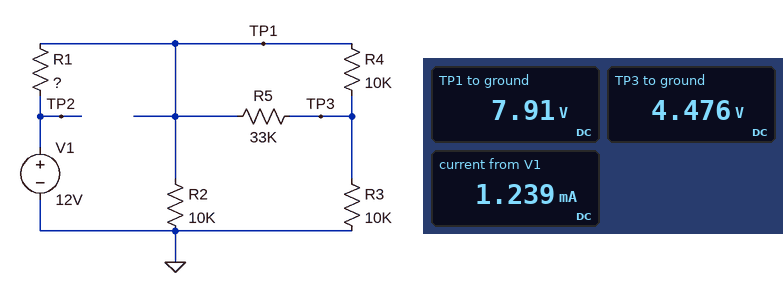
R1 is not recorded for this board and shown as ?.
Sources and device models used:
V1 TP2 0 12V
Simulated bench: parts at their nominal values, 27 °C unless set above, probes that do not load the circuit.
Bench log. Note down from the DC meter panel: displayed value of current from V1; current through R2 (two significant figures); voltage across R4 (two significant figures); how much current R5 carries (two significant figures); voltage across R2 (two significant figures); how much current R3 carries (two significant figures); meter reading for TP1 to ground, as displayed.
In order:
1.239 mA
790 µA
3.4 V
100 µA
7.9 V
450 µA
7.91 V
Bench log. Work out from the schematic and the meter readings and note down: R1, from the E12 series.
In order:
3.3 kΩ
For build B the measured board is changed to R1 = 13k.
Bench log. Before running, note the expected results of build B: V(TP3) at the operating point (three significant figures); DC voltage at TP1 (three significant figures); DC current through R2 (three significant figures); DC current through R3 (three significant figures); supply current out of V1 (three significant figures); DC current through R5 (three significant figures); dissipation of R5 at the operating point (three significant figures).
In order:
2.24 V
3.95 V
395 µA
224 µA
619 µA
52.0 µA
89.3 µW
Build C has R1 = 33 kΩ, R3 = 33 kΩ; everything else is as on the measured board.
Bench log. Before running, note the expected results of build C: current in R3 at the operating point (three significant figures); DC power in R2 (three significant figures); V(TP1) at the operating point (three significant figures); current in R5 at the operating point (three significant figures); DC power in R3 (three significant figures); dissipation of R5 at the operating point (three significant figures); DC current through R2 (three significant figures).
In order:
57.7 µA
551 µW
2.35 V
13.4 µA
110 µW
5.95 µW
235 µA
